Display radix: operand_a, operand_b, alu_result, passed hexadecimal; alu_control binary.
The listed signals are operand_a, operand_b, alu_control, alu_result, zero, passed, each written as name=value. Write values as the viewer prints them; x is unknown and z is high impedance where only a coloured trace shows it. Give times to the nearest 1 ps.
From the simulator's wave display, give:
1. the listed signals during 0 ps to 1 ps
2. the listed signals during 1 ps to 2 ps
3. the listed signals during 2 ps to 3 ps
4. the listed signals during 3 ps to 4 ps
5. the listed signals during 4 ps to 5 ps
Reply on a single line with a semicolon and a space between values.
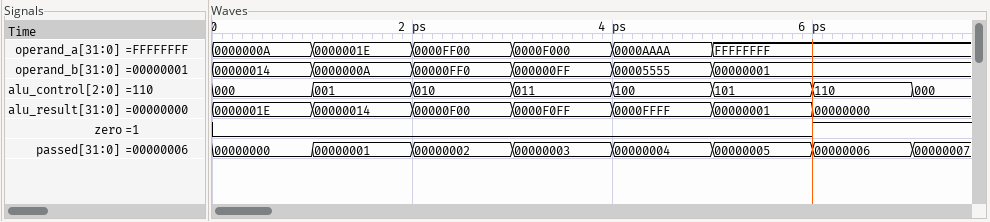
operand_a=0000000A, operand_b=00000014, alu_control=000, alu_result=0000001E, zero=0, passed=00000000; operand_a=0000001E, operand_b=0000000A, alu_control=001, alu_result=00000014, zero=0, passed=00000001; operand_a=0000FF00, operand_b=00000FF0, alu_control=010, alu_result=00000F00, zero=0, passed=00000002; operand_a=0000F000, operand_b=000000FF, alu_control=011, alu_result=0000F0FF, zero=0, passed=00000003; operand_a=0000AAAA, operand_b=00005555, alu_control=100, alu_result=0000FFFF, zero=0, passed=00000004
